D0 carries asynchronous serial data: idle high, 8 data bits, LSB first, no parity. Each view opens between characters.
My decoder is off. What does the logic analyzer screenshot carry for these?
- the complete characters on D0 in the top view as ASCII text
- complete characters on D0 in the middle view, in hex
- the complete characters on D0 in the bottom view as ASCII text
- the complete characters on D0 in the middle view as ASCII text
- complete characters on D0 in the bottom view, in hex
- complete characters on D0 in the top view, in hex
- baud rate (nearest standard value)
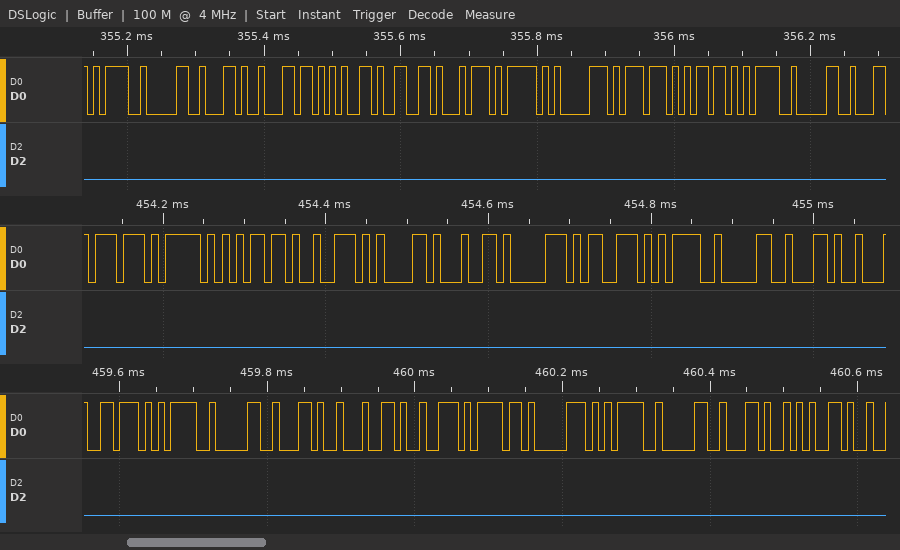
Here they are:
"=0,left_pwm=0"
77, 5F, 6D, 72, 61, 64, 70, 73, 3D, 30, 2C
"v=0,drop=0,e"
"w_mradps=0,"
76, 3D, 30, 2C, 64, 72, 6F, 70, 3D, 30, 2C, 65
3D, 30, 2C, 6C, 65, 66, 74, 5F, 70, 77, 6D, 3D, 30
115200 baud
